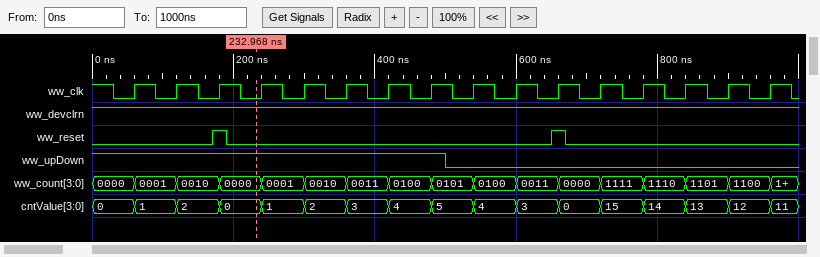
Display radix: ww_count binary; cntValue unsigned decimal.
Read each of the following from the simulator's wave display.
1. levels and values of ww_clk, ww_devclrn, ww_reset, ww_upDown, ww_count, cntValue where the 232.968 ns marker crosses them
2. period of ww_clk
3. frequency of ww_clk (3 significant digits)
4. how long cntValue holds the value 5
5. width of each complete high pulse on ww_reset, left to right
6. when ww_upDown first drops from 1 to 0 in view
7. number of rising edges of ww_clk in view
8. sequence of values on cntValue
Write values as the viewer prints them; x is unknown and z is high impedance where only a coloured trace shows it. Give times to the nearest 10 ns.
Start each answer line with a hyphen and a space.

- ww_clk=0, ww_devclrn=1, ww_reset=0, ww_upDown=1, ww_count=0000, cntValue=0
- 60 ns
- 16.7 MHz
- 60 ns
- 20 ns, 20 ns
- 500 ns
- 16
- 0, 1, 2, 0, 1, 2, 3, 4, 5, 4, 3, 0, 15, 14, 13, 12, 11
